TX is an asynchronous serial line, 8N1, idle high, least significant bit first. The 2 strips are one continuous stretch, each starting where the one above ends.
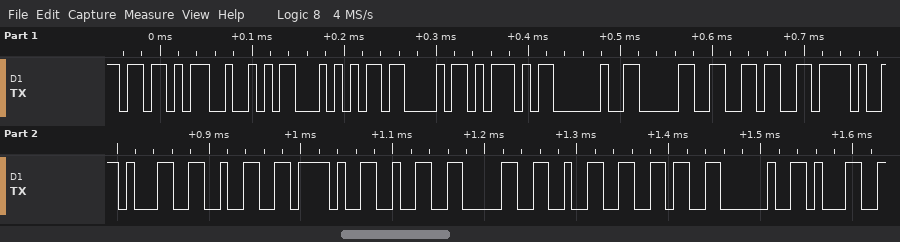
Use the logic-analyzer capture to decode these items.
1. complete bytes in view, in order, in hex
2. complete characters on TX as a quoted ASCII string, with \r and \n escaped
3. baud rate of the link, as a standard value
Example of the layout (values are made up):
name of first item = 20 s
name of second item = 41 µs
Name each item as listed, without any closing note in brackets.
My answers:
complete bytes in view, in order, in hex = 0x5B 0x52 0x54 0x43 0x5D 0x20 0x30 0x36 0x2F 0x31 0x32 0x2F 0x32 0x30 0x32 0x36 0x20 0x31
complete characters on TX as a quoted ASCII string, with \r and \n escaped = "[RTC] 06/12/2026 1"
baud rate of the link, as a standard value = 115200 baud
